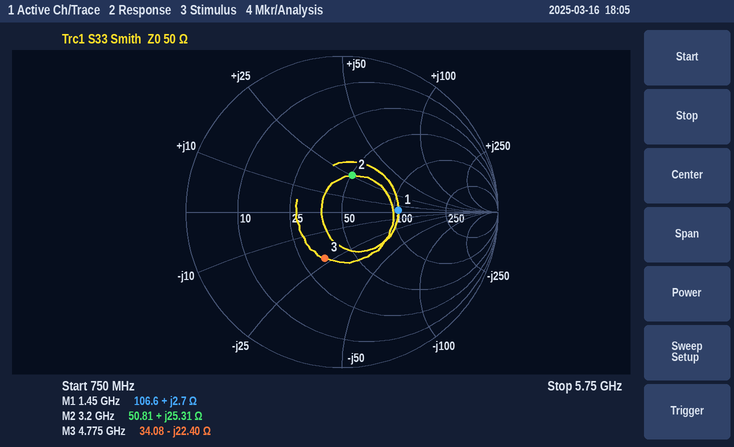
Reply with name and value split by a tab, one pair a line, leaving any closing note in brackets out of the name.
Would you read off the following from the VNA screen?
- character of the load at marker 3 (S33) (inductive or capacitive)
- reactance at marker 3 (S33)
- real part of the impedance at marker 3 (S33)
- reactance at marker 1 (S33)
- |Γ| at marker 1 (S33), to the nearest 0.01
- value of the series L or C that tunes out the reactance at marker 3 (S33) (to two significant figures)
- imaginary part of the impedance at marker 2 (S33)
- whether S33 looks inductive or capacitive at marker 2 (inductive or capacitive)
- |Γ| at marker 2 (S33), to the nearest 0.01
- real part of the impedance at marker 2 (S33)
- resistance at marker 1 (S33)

character of the load at marker 3 (S33)	capacitive
reactance at marker 3	-22.40 Ω
real part of the impedance at marker 3	34.08 Ω
reactance at marker 1	+2.7 Ω
|Γ| at marker 1 (S33), to the nearest 0.01	0.36
value of the series L or C that tunes out the reactance at marker 3 (S33)	750 pH
imaginary part of the impedance at marker 2	+25.31 Ω
whether S33 looks inductive or capacitive at marker 2	inductive
|Γ| at marker 2 (S33), to the nearest 0.01	0.24
real part of the impedance at marker 2	50.81 Ω
resistance at marker 1	106.6 Ω
